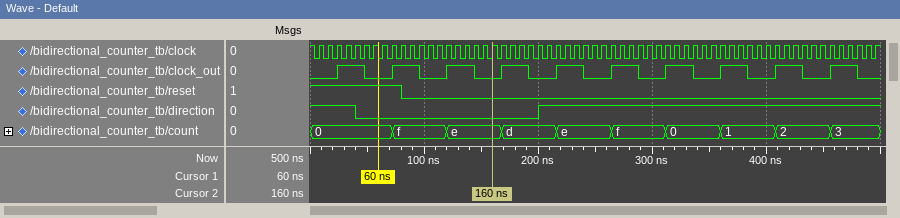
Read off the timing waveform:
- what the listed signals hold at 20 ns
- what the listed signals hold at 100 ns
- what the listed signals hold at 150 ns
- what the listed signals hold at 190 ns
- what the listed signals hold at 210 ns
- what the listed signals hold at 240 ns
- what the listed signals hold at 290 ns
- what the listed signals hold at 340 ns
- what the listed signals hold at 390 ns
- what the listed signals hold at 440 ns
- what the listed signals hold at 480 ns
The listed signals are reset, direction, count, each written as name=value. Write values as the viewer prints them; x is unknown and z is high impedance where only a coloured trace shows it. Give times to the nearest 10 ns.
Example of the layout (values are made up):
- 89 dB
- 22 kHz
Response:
- reset=1, direction=1, count=0
- reset=0, direction=0, count=f
- reset=0, direction=0, count=e
- reset=0, direction=0, count=d
- reset=0, direction=1, count=d
- reset=0, direction=1, count=e
- reset=0, direction=1, count=f
- reset=0, direction=1, count=0
- reset=0, direction=1, count=1
- reset=0, direction=1, count=2
- reset=0, direction=1, count=3
